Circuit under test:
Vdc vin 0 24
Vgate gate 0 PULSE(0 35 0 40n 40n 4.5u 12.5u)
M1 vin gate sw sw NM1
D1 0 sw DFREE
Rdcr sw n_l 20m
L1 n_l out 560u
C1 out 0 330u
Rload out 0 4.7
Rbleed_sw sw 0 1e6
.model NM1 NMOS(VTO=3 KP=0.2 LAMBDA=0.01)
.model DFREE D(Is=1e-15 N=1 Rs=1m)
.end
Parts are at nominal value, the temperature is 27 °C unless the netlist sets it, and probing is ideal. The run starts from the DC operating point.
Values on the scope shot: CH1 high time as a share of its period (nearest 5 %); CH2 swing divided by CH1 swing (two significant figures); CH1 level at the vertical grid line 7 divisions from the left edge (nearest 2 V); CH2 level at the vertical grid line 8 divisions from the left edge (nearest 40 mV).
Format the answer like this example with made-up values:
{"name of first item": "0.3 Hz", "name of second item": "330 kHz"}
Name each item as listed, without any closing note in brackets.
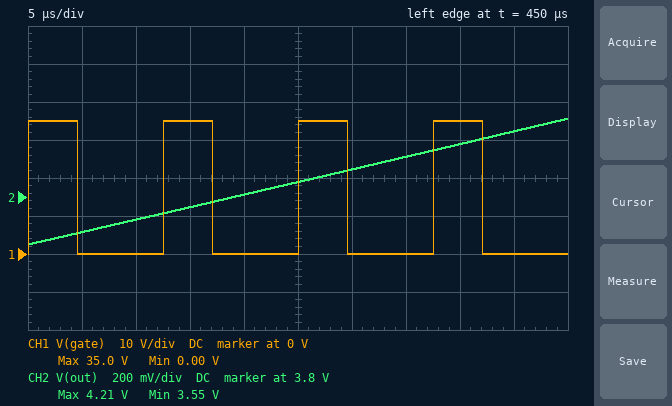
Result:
{"CH1 high time as a share of its period": "35 %", "CH2 swing divided by CH1 swing": "0.019", "CH1 level at the vertical grid line 7 divisions from the left edge": "0 V", "CH2 level at the vertical grid line 8 divisions from the left edge": "4.08 V"}
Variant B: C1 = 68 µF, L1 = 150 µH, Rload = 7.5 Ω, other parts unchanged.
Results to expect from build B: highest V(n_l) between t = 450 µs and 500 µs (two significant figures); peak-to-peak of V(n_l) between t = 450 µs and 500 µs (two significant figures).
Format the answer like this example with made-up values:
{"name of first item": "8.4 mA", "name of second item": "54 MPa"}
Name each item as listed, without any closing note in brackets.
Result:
{"highest V(n_l) between t = 450 µs and 500 µs": "24 V", "peak-to-peak of V(n_l) between t = 450 µs and 500 µs": "25 V"}
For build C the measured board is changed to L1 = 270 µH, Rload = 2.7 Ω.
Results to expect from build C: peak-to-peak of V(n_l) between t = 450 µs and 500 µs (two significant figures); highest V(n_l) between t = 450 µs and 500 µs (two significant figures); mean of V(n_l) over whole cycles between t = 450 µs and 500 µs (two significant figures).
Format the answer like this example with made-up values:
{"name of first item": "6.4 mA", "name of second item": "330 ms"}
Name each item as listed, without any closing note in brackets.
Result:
{"peak-to-peak of V(n_l) between t = 450 µs and 500 µs": "21 V", "highest V(n_l) between t = 450 µs and 500 µs": "20 V", "mean of V(n_l) over whole cycles between t = 450 µs and 500 µs": "6.5 V"}
